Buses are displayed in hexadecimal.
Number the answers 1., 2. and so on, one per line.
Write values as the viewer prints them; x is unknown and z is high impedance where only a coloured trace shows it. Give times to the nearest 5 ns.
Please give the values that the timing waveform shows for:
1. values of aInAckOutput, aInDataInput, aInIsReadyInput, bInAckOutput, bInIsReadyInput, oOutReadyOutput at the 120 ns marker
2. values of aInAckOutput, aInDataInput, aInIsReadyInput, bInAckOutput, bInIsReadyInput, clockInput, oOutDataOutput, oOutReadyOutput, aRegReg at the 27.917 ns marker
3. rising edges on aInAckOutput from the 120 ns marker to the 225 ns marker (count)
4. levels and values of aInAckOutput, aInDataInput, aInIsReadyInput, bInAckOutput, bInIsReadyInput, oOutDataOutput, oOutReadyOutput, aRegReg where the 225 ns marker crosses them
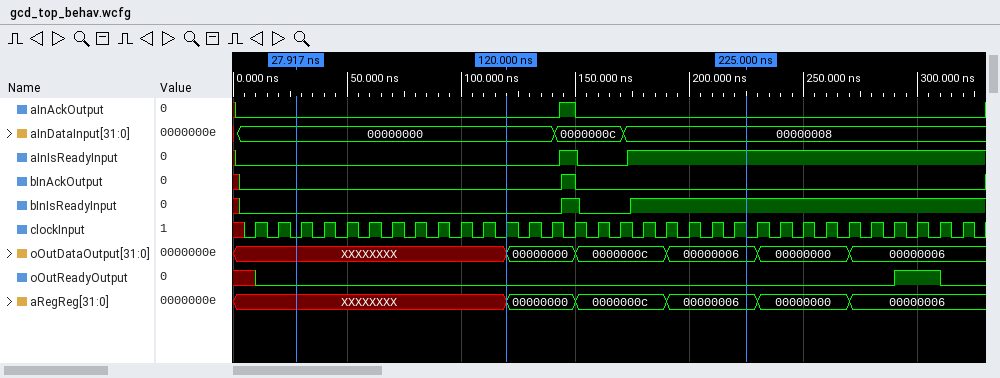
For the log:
1. aInAckOutput=0, aInDataInput=00000000, aInIsReadyInput=0, bInAckOutput=0, bInIsReadyInput=0, oOutReadyOutput=0
2. aInAckOutput=0, aInDataInput=00000000, aInIsReadyInput=0, bInAckOutput=0, bInIsReadyInput=0, clockInput=0, oOutDataOutput=XXXXXXXX, oOutReadyOutput=0, aRegReg=XXXXXXXX
3. 1
4. aInAckOutput=0, aInDataInput=00000008, aInIsReadyInput=1, bInAckOutput=0, bInIsReadyInput=1, oOutDataOutput=00000006, oOutReadyOutput=0, aRegReg=00000006
